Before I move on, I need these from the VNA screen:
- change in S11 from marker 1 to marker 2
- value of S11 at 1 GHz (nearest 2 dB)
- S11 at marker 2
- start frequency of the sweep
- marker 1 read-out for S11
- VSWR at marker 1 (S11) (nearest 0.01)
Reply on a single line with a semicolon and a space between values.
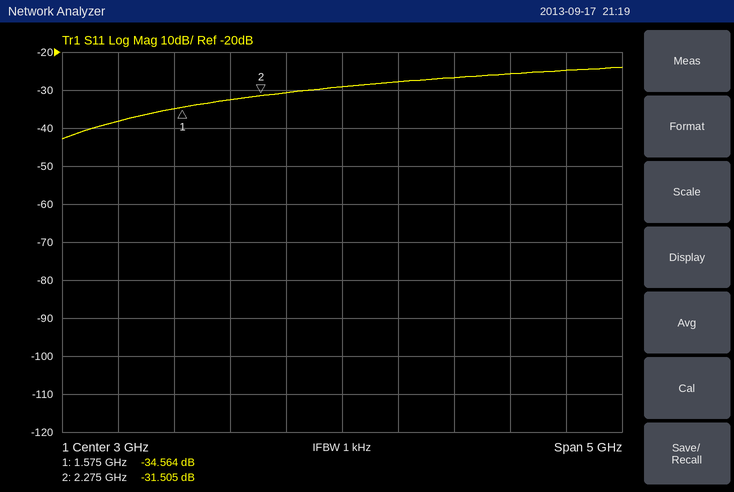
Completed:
3.059 dB; -38 dB; -31.505 dB; 500 MHz; -34.564 dB; 1.04
